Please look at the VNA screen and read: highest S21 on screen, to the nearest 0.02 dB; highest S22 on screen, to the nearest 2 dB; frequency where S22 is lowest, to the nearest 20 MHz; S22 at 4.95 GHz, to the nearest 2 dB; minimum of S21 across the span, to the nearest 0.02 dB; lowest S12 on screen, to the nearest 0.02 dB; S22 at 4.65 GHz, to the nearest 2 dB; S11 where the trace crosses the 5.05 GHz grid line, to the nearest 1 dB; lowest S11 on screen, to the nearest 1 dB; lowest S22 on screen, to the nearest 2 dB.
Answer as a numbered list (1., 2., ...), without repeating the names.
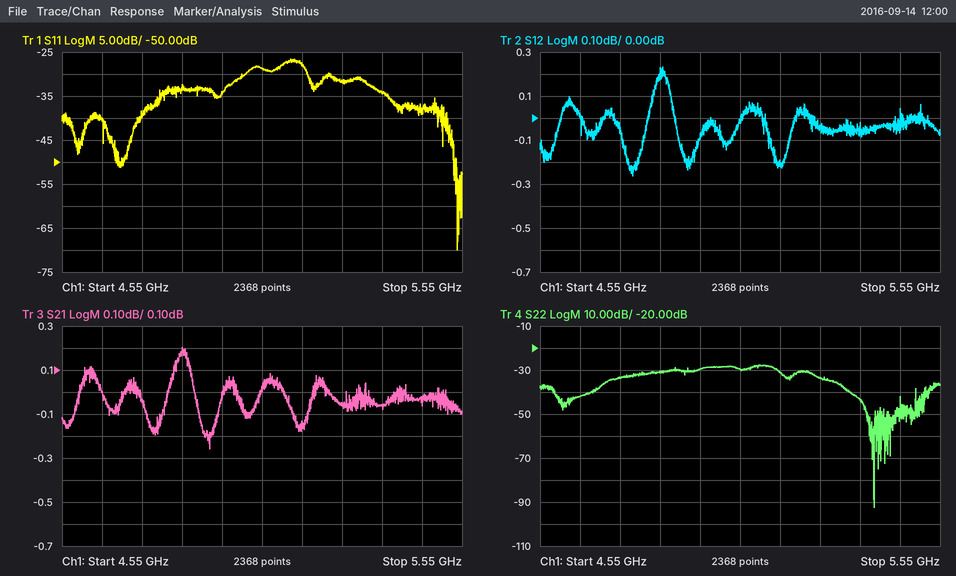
1. 0.20 dB
2. -28 dB
3. 5.38 GHz
4. -30 dB
5. -0.26 dB
6. -0.26 dB
7. -42 dB
8. -29 dB
9. -70 dB
10. -92 dB
